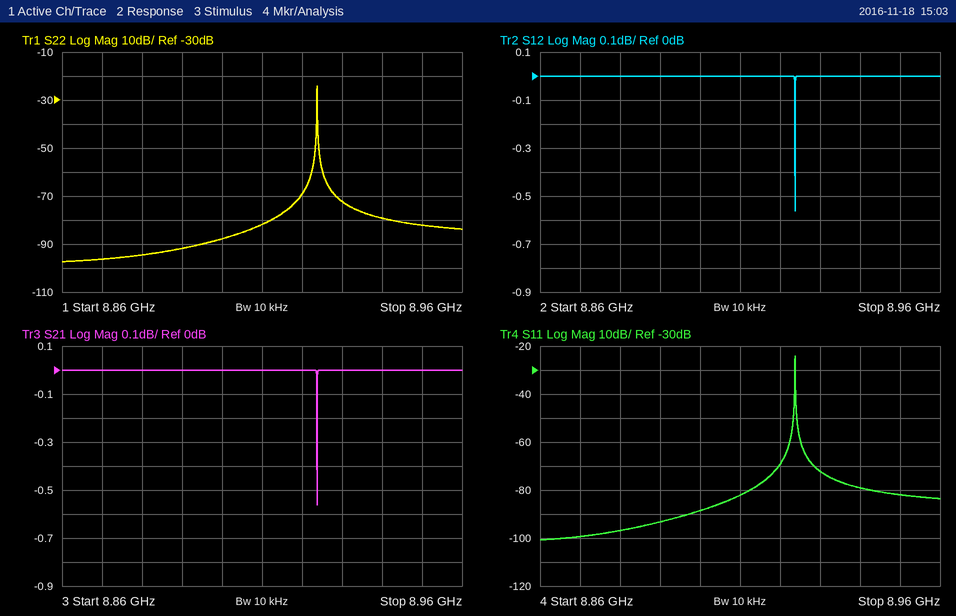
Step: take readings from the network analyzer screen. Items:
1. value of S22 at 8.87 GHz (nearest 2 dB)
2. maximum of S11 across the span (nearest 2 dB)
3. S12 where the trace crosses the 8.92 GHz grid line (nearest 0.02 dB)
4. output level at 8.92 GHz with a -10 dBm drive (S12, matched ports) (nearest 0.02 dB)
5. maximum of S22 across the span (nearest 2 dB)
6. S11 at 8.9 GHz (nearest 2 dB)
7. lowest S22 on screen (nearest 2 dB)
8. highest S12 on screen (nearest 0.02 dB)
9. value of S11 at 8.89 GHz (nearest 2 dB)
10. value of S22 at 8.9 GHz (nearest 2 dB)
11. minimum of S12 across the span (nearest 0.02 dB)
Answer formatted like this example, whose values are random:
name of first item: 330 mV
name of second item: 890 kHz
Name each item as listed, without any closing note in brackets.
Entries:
value of S22 at 8.87 GHz: -96 dB
maximum of S11 across the span: -24 dB
S12 where the trace crosses the 8.92 GHz grid line: 0.00 dB
output level at 8.92 GHz with a -10 dBm drive (S12, matched ports): -10.00 dBm
maximum of S22 across the span: -24 dB
S11 at 8.9 GHz: -88 dB
lowest S22 on screen: -98 dB
highest S12 on screen: 0.00 dB
value of S11 at 8.89 GHz: -94 dB
value of S22 at 8.9 GHz: -88 dB
minimum of S12 across the span: -0.56 dB
